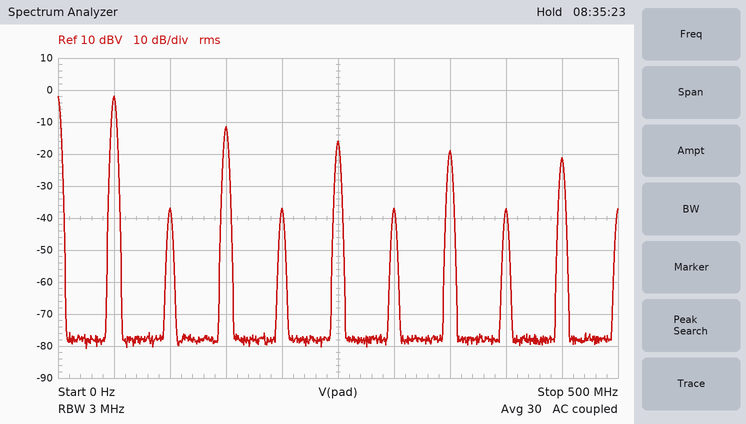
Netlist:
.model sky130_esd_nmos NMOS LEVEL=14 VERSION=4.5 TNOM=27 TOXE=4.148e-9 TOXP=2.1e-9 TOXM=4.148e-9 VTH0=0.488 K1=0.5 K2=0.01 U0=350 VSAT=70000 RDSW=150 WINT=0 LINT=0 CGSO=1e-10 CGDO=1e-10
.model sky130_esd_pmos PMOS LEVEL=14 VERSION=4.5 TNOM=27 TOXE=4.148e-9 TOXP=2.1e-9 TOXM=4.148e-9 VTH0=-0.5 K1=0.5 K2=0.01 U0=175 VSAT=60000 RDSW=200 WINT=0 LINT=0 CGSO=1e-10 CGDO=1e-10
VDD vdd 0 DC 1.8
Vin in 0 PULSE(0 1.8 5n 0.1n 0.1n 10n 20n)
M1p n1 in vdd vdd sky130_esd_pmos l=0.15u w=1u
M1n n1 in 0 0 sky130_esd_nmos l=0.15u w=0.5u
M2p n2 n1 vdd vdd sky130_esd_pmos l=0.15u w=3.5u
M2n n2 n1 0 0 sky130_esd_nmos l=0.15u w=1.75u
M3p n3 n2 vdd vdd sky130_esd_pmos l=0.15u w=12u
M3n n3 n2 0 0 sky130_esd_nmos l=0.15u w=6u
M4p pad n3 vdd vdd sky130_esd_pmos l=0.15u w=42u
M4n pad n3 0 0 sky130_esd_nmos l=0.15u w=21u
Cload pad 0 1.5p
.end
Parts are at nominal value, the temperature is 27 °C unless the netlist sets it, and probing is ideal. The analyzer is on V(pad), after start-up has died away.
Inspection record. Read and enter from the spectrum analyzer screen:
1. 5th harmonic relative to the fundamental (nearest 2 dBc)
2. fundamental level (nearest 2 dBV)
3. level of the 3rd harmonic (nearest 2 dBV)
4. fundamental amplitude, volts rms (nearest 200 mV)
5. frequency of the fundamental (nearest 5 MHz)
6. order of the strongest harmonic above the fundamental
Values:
-14 dBc
-2 dBV
-12 dBV
800 mV
50 MHz
3
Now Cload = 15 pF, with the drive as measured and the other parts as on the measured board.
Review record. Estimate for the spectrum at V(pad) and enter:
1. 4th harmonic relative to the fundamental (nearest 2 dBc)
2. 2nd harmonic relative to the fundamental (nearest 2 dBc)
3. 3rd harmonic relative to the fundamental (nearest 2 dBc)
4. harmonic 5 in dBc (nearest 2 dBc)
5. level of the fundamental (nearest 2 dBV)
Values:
-30 dBc
-28 dBc
-10 dBc
-18 dBc
-2 dBV
